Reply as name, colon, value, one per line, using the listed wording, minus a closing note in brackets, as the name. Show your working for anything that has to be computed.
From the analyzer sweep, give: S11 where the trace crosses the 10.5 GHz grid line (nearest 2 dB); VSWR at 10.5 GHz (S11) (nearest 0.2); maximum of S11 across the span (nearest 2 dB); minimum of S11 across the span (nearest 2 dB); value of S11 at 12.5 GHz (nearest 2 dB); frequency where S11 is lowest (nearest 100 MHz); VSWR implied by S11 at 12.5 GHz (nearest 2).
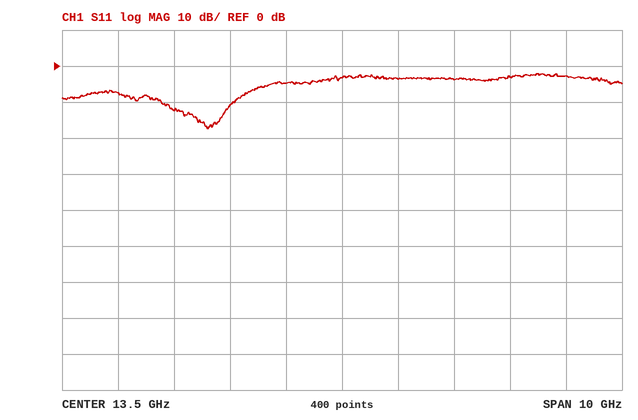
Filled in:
S11 where the trace crosses the 10.5 GHz grid line: -12 dB
VSWR at 10.5 GHz (S11): |Γ| = 10^(-12/20) = 0.2512; VSWR = (1 + 0.2512)/(1 − 0.2512) ≈ 1.67, so 1.6 to the nearest 0.2
maximum of S11 across the span: -2 dB
minimum of S11 across the span: -18 dB
value of S11 at 12.5 GHz: -4 dB
frequency where S11 is lowest: 11.1 GHz
VSWR implied by S11 at 12.5 GHz: |Γ| = 10^(-4/20) = 0.6310; VSWR = (1 + 0.6310)/(1 − 0.6310) ≈ 4
